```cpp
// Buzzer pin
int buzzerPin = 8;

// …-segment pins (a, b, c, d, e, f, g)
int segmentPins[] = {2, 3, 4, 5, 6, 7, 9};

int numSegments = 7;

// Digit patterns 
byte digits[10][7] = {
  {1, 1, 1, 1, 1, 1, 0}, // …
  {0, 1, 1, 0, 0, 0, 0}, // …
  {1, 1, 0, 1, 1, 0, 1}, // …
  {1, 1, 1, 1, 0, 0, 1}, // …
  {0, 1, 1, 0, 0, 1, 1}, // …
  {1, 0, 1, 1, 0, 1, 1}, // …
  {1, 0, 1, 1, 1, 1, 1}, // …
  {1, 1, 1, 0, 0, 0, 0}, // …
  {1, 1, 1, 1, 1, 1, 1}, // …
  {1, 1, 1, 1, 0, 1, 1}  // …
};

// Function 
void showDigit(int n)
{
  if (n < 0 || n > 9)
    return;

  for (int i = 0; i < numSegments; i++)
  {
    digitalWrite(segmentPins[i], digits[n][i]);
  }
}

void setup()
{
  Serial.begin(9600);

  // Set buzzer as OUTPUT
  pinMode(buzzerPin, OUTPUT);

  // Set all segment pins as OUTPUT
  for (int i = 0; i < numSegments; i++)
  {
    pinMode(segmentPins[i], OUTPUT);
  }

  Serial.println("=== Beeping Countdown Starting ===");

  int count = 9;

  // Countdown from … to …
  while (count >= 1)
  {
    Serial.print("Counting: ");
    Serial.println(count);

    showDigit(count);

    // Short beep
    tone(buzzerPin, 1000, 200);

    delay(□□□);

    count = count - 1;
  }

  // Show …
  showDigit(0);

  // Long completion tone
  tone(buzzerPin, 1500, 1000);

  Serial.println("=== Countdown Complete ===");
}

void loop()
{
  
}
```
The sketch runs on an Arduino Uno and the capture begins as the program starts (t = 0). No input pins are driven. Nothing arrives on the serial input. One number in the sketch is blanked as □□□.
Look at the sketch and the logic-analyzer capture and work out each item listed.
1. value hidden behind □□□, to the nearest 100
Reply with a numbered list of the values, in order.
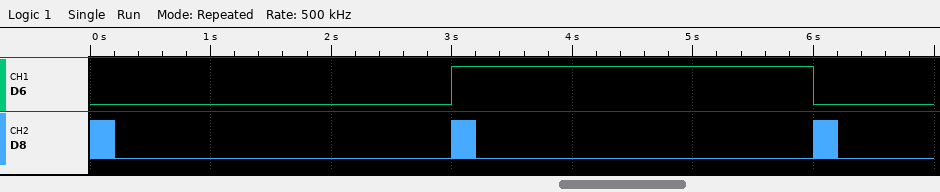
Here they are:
1. 3000
